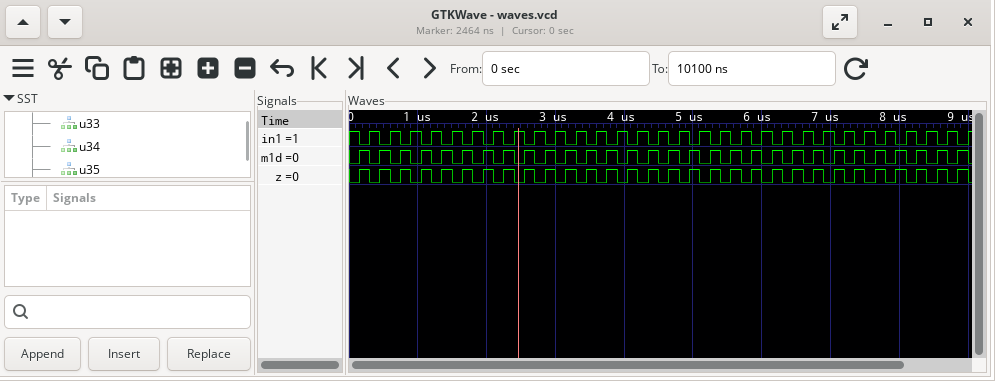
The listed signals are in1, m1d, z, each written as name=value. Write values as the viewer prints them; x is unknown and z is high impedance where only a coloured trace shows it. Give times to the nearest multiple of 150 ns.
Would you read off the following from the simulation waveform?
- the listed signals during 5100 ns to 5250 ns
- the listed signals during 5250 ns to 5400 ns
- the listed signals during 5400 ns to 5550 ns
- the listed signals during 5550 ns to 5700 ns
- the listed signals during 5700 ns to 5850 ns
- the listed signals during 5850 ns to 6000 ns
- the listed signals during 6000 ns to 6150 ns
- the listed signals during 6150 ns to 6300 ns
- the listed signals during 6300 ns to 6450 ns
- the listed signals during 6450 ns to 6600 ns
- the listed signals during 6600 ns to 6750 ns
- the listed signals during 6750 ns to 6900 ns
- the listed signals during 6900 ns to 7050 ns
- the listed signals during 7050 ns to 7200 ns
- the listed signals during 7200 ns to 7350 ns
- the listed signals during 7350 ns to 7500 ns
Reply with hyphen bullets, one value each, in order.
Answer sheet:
- in1=1, m1d=0, z=0
- in1=0, m1d=1, z=1
- in1=1, m1d=0, z=0
- in1=0, m1d=1, z=1
- in1=1, m1d=0, z=0
- in1=0, m1d=1, z=1
- in1=1, m1d=0, z=0
- in1=0, m1d=1, z=1
- in1=1, m1d=0, z=0
- in1=0, m1d=1, z=1
- in1=1, m1d=0, z=0
- in1=0, m1d=1, z=1
- in1=1, m1d=0, z=0
- in1=0, m1d=1, z=1
- in1=1, m1d=0, z=0
- in1=0, m1d=1, z=1
